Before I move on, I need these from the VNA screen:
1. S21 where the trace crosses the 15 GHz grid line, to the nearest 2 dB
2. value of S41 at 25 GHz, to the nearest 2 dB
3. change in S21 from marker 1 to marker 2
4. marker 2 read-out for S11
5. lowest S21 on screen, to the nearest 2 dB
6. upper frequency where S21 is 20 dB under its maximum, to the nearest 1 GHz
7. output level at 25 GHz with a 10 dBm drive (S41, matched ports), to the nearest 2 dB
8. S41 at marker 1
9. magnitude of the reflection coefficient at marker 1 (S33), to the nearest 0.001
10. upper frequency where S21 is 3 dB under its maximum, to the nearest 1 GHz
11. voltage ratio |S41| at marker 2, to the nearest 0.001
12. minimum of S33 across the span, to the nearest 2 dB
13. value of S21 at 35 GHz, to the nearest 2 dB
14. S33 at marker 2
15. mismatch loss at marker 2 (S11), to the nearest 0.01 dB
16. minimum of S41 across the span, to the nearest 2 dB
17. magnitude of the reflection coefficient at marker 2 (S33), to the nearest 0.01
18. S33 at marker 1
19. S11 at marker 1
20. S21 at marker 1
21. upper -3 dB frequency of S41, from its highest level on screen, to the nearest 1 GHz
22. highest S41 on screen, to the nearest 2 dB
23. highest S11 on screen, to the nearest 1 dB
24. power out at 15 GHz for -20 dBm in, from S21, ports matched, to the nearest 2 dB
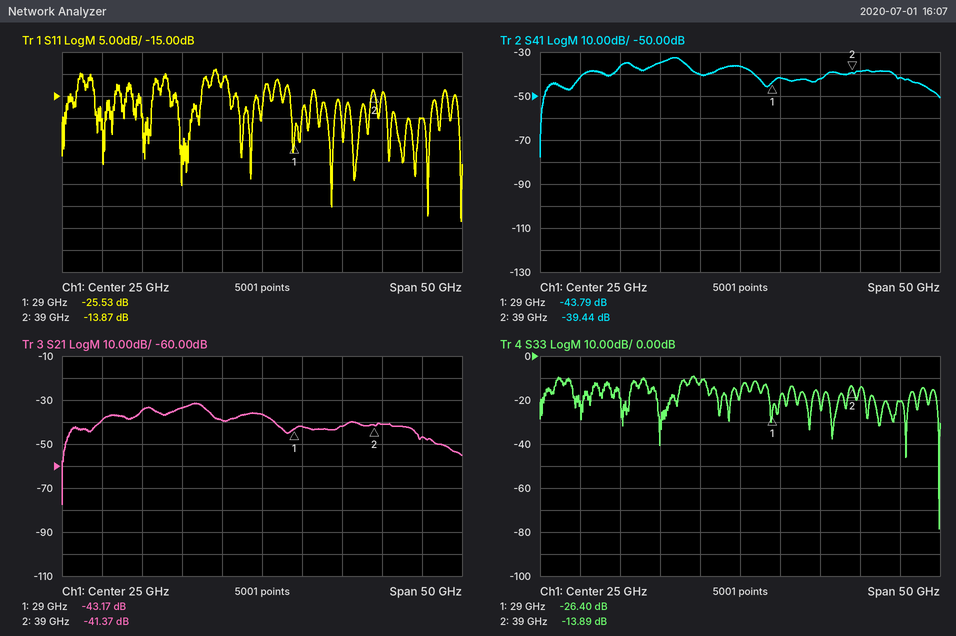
-34 dB
-36 dB
1.80 dB
-13.87 dB
-78 dB
48 GHz
-26 dBm
-43.79 dB
0.048
18 GHz
0.011
-78 dB
-42 dB
-13.89 dB
0.18 dB
-78 dB
0.20
-26.40 dB
-25.53 dB
-43.17 dB
18 GHz
-32 dB
-9 dB
-54 dBm
